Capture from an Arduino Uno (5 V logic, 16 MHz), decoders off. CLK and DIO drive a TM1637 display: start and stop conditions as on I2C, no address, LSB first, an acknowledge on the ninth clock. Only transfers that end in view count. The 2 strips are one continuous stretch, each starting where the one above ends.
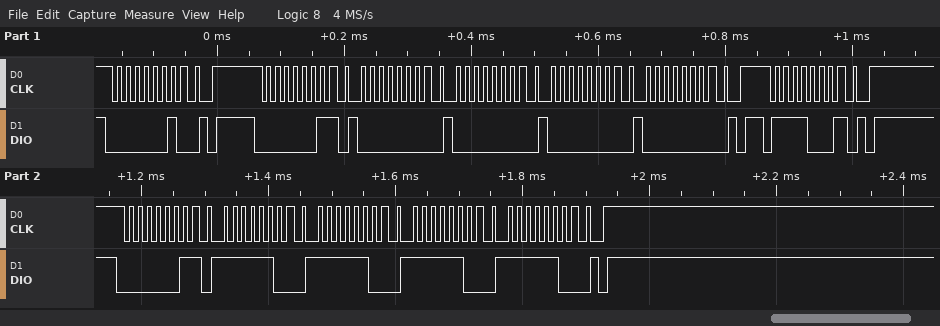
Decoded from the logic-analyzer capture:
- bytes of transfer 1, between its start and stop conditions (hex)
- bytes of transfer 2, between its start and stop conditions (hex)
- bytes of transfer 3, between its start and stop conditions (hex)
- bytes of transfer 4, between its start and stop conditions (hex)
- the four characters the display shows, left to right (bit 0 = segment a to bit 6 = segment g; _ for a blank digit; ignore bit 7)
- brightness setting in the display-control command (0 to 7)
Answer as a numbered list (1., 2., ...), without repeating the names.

1. 40
2. C0 00 00 00 00
3. 8F
4. C0 3F 3F 3F 3F
5. 0000
6. 7
